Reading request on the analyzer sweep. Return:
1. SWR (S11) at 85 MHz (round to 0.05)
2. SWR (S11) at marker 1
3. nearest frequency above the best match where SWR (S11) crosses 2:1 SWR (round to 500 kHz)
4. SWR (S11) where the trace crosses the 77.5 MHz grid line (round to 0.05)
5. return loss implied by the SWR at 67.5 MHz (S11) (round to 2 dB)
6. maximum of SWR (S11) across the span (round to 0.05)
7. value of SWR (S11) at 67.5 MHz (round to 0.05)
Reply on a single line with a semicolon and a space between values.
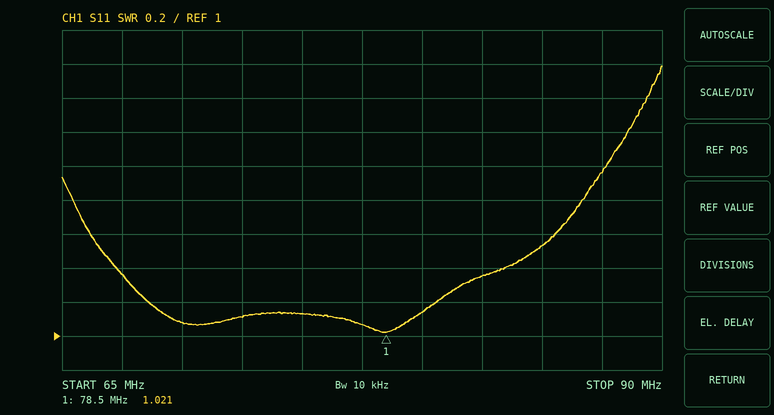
1.55; 1.021; 87.5 MHz; 1.05; 16 dB; 2.60; 1.35
